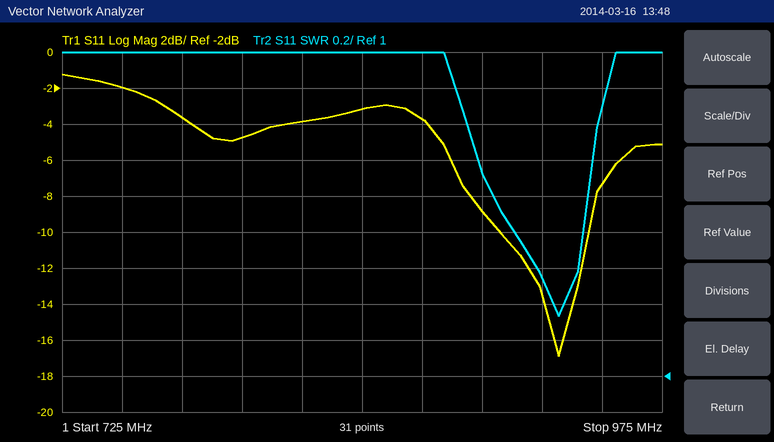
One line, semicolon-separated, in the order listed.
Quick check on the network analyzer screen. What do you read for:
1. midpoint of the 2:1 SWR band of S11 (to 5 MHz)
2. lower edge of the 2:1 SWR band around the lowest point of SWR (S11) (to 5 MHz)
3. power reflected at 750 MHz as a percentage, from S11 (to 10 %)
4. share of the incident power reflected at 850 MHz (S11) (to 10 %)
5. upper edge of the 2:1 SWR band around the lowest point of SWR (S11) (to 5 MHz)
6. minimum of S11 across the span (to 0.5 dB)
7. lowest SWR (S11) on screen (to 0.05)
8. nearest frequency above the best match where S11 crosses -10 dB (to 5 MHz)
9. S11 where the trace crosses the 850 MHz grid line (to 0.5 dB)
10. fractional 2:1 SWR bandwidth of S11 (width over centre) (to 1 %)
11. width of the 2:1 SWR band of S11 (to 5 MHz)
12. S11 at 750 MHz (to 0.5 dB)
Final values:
925 MHz; 905 MHz; 60 %; 50 %; 945 MHz; -17.0 dB; 1.35; 945 MHz; -3.0 dB; 4 %; 40 MHz; -2.0 dB
